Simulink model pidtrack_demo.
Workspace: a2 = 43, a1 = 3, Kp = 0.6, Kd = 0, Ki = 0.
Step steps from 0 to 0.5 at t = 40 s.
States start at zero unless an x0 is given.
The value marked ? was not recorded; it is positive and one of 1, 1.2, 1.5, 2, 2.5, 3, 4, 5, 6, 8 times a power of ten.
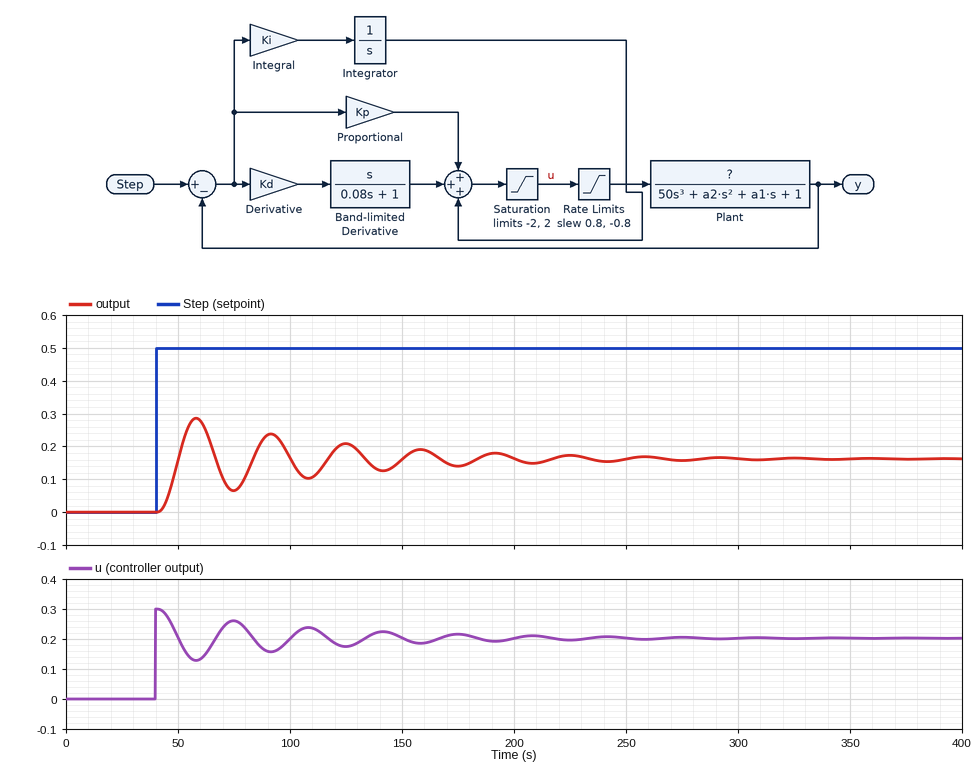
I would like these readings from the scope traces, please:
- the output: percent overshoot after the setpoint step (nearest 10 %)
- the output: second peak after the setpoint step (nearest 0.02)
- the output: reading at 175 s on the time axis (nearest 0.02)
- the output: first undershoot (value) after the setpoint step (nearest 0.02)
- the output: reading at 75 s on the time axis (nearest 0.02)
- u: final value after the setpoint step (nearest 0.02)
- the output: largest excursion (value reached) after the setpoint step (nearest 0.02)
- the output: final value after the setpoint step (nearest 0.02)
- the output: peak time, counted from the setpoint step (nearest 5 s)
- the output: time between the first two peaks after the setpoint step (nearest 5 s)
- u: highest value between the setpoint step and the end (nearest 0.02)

80 %
0.24
0.14
0.06
0.06
0.20
0.28
0.16
20 s
35 s
0.30
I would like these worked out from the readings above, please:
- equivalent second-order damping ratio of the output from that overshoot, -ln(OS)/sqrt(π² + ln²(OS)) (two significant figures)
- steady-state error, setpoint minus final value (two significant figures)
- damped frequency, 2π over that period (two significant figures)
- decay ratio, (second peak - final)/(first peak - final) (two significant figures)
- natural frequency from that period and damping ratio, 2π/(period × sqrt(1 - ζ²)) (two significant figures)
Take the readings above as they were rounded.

0.071
0.34
0.18 rad/s
0.67
0.18 rad/s
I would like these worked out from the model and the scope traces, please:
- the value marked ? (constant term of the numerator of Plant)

0.8
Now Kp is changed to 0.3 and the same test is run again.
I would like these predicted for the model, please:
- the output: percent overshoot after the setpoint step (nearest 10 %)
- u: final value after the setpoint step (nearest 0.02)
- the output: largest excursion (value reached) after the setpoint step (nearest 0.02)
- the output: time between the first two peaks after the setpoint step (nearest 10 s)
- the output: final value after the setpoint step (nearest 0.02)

70 %
0.12
0.16
40 s
0.10
